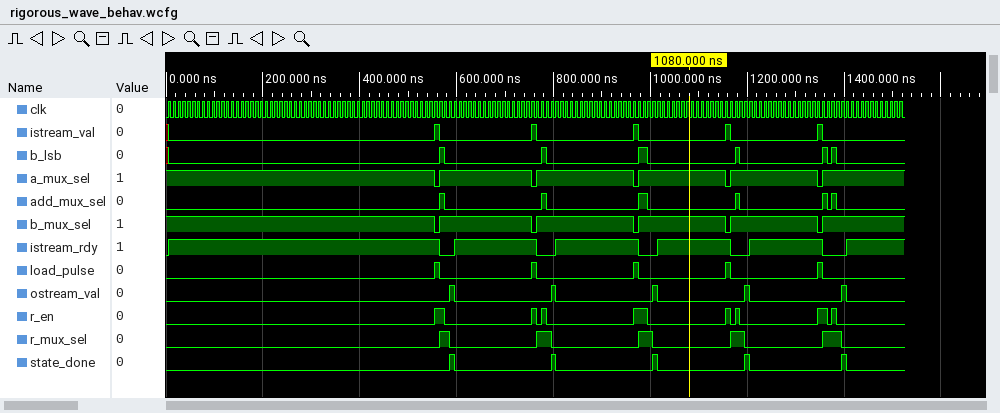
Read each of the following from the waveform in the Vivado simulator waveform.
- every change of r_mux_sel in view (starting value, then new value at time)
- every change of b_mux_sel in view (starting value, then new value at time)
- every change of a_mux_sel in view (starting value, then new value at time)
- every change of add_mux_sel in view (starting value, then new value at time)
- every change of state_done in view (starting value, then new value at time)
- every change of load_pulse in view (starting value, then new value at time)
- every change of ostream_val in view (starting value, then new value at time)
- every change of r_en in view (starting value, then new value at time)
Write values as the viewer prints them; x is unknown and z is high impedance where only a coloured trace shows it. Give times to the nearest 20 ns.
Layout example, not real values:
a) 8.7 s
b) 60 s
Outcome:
a) 0, 1 at 560 ns, 0 at 580 ns, 1 at 760 ns, 0 at 800 ns, 1 at 980 ns, 0 at 1000 ns, 1 at 1160 ns, 0 at 1200 ns, 1 at 1360 ns, 0 at 1400 ns
b) 1, 0 at 560 ns, 1 at 560 ns, 0 at 760 ns, 1 at 760 ns, 0 at 960 ns, 1 at 980 ns, 0 at 1160 ns, 1 at 1160 ns, 0 at 1340 ns, 1 at 1360 ns
c) 1, 0 at 560 ns, 1 at 560 ns, 0 at 760 ns, 1 at 760 ns, 0 at 960 ns, 1 at 980 ns, 0 at 1160 ns, 1 at 1160 ns, 0 at 1340 ns, 1 at 1360 ns
d) 0, 1 at 560 ns, 0 at 580 ns, 1 at 780 ns, 0 at 780 ns, 1 at 980 ns, 0 at 1000 ns, 1 at 1180 ns, 0 at 1180 ns, 1 at 1360 ns, 0 at 1360 ns, 1 at 1380 ns, 0 at 1380 ns
e) 0, 1 at 580 ns, 0 at 600 ns, 1 at 800 ns, 0 at 800 ns, 1 at 1000 ns, 0 at 1020 ns, 1 at 1200 ns, 0 at 1200 ns, 1 at 1400 ns, 0 at 1400 ns
f) 0, 1 at 560 ns, 0 at 560 ns, 1 at 760 ns, 0 at 760 ns, 1 at 960 ns, 0 at 980 ns, 1 at 1160 ns, 0 at 1160 ns, 1 at 1340 ns, 0 at 1360 ns
g) 0, 1 at 580 ns, 0 at 600 ns, 1 at 800 ns, 0 at 800 ns, 1 at 1000 ns, 0 at 1020 ns, 1 at 1200 ns, 0 at 1200 ns, 1 at 1400 ns, 0 at 1400 ns
h) 0, 1 at 560 ns, 0 at 580 ns, 1 at 760 ns, 0 at 760 ns, 1 at 780 ns, 0 at 780 ns, 1 at 960 ns, 0 at 1000 ns, 1 at 1160 ns, 0 at 1160 ns, 1 at 1180 ns, 0 at 1180 ns, 1 at 1340 ns, 0 at 1360 ns, 1 at 1380 ns, 0 at 1380 ns
